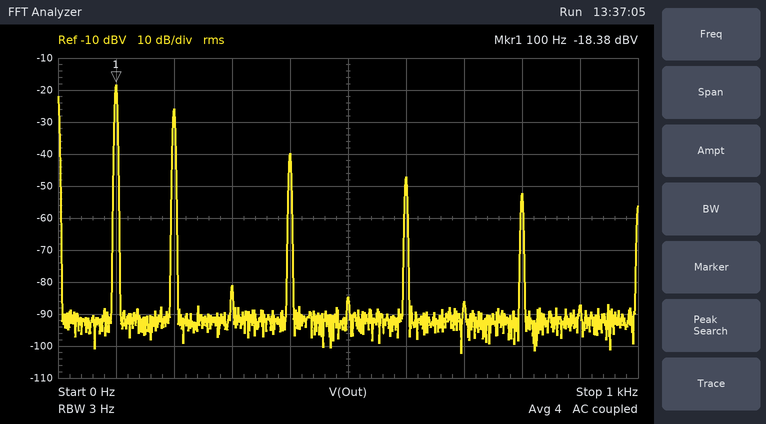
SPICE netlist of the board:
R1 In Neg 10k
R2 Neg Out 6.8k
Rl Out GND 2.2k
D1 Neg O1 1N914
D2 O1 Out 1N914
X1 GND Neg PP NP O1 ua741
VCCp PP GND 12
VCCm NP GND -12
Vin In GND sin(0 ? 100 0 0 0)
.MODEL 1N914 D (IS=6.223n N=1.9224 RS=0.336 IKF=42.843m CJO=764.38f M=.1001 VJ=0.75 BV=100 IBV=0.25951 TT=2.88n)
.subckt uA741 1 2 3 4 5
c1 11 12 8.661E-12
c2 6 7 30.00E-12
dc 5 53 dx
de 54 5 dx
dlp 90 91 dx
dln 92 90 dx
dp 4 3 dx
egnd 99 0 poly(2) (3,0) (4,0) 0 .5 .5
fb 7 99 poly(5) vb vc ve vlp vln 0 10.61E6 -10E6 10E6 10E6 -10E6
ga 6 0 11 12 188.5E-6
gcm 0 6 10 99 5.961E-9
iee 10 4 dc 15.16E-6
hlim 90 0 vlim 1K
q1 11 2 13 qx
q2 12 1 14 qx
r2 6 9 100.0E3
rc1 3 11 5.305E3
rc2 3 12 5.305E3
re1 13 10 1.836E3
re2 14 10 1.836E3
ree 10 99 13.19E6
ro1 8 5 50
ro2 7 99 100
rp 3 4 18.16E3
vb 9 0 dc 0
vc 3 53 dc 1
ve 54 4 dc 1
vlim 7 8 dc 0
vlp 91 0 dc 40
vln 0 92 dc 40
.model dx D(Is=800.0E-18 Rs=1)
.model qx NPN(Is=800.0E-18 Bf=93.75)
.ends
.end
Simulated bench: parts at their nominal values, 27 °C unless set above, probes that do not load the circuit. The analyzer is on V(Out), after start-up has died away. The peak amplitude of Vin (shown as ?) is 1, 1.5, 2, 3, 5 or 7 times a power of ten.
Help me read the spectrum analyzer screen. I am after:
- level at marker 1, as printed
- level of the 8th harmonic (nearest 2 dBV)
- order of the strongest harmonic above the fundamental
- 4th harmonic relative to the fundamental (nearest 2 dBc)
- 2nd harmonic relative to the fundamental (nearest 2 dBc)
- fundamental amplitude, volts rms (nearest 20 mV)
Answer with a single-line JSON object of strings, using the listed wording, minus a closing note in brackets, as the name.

{"level at marker 1, as printed": "-18.38 dBV", "level of the 8th harmonic": "-52 dBV", "order of the strongest harmonic above the fundamental": "2", "4th harmonic relative to the fundamental": "-22 dBc", "2nd harmonic relative to the fundamental": "-8 dBc", "fundamental amplitude, volts rms": "120 mV"}
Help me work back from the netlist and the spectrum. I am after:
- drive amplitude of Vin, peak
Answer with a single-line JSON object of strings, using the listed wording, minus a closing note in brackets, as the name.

{"drive amplitude of Vin, peak": "500 mV"}
